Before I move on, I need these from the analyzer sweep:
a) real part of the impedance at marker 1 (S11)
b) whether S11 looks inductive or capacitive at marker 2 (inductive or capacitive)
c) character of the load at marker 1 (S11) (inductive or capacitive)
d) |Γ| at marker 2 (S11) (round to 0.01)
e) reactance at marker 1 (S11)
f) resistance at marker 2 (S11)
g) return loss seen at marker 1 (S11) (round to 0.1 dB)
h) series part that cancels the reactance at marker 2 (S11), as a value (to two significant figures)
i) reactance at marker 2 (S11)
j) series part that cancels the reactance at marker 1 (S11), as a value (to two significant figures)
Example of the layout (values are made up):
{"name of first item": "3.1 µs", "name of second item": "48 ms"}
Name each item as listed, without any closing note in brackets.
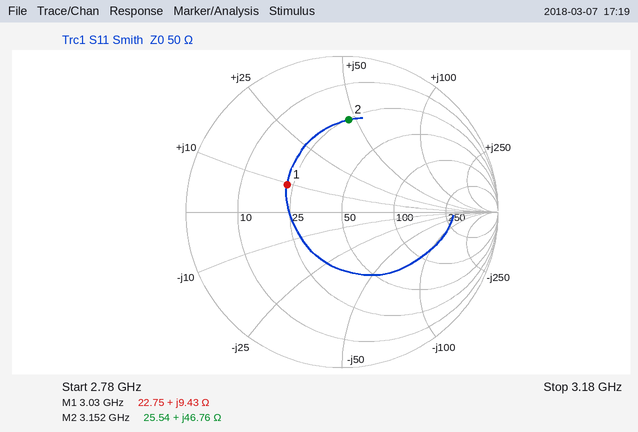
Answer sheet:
{"real part of the impedance at marker 1": "22.75 Ω", "whether S11 looks inductive or capacitive at marker 2": "inductive", "character of the load at marker 1 (S11)": "inductive", "|Γ| at marker 2 (S11)": "0.59", "reactance at marker 1": "+9.43 Ω", "resistance at marker 2": "25.54 Ω", "return loss seen at marker 1 (S11)": "8.1 dB", "series part that cancels the reactance at marker 2 (S11), as a value": "1.1 pF", "reactance at marker 2": "+46.76 Ω", "series part that cancels the reactance at marker 1 (S11), as a value": "5.6 pF"}
